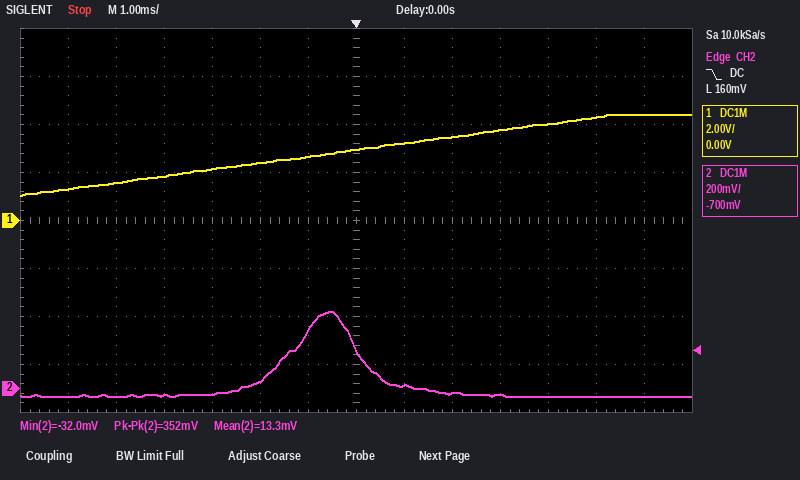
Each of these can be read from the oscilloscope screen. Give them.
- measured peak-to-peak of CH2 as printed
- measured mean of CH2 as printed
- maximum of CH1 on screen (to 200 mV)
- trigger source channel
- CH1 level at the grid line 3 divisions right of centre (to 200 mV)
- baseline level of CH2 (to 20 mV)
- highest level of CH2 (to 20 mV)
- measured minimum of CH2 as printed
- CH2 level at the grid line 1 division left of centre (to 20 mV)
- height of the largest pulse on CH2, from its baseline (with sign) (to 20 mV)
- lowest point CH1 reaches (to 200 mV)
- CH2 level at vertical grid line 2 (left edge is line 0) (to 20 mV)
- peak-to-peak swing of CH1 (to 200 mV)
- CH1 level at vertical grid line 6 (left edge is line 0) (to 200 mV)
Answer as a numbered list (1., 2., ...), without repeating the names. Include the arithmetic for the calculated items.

1. 352 mV
2. 13.3 mV
3. 4.4 V
4. CH2
5. 3.8 V
6. -40 mV
7. 320 mV
8. -32.0 mV
9. 240 mV
10. 320 mV − (-40 mV) = +360 mV
11. 1.0 V
12. -40 mV
13. 4.4 V − (1.0 V) = 3.4 V
14. 2.6 V
